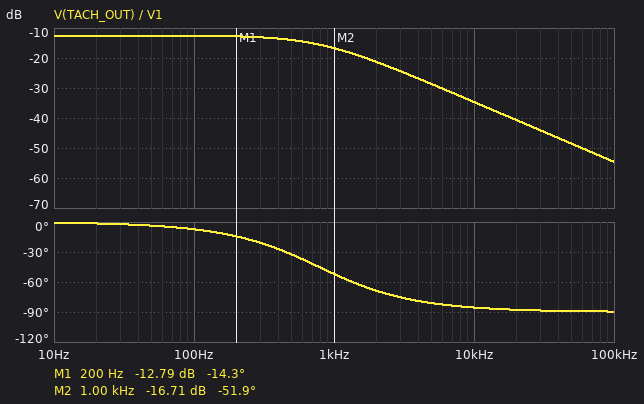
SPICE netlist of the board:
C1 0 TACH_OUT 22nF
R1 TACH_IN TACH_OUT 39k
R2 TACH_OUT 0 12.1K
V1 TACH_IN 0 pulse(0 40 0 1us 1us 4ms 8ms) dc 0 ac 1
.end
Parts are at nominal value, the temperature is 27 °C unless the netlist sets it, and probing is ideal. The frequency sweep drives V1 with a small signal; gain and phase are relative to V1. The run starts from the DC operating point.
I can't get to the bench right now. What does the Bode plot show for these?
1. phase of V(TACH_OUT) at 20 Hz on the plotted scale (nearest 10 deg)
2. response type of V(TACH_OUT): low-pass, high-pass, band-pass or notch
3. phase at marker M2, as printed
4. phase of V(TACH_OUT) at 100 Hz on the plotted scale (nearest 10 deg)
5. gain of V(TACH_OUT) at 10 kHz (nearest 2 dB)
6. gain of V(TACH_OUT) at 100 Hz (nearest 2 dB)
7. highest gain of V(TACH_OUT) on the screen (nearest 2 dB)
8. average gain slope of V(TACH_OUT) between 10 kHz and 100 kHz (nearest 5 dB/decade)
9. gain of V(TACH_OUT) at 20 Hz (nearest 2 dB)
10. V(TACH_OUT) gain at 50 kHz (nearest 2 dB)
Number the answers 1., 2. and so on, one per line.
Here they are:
1. 0 deg
2. low-pass
3. -51.9 deg
4. -10 deg
5. -34 dB
6. -12 dB
7. -12 dB
8. -20 dB/decade
9. -12 dB
10. -48 dB
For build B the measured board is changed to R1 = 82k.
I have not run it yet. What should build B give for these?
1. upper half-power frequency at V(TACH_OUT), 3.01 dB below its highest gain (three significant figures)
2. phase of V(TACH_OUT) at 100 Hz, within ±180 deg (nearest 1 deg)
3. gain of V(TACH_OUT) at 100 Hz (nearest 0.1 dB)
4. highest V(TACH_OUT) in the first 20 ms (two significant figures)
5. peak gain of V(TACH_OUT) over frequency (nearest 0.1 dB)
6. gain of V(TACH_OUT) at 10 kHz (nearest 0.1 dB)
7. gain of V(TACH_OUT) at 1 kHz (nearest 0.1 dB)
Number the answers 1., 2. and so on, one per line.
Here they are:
1. 686 Hz
2. -8 deg
3. -17.9 dB
4. 5.1 V
5. -17.8 dB
6. -41.1 dB
7. -22.8 dB
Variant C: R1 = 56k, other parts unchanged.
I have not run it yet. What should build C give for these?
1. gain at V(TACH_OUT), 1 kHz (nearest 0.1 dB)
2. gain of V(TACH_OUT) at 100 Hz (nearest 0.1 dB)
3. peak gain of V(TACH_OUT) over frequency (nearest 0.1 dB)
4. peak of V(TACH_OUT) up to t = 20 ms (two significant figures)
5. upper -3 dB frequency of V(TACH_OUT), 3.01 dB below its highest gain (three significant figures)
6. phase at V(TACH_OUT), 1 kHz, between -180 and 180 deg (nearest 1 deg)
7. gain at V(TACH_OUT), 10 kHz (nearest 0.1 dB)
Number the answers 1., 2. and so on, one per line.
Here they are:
1. -19.6 dB
2. -15.1 dB
3. -15.0 dB
4. 7.1 V
5. 727 Hz
6. -54 deg
7. -37.8 dB
